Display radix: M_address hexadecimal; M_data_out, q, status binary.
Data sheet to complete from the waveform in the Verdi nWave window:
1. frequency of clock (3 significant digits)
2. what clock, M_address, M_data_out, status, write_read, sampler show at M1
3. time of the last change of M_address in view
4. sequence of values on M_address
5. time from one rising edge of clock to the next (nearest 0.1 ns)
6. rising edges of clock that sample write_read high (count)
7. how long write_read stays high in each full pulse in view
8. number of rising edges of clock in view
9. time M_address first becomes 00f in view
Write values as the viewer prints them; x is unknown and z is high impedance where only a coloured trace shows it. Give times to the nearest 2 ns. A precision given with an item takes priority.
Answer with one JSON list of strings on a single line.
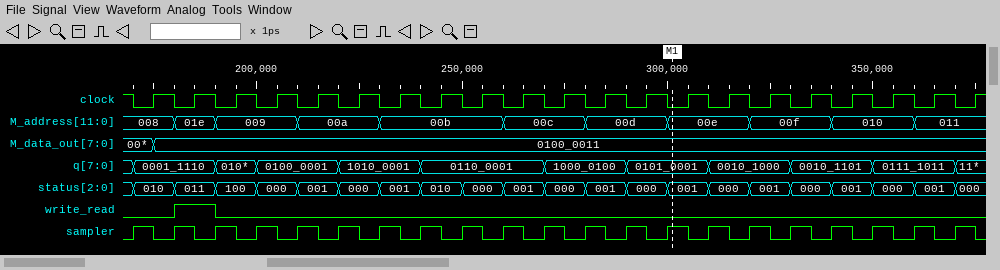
["100 MHz", "clock=0, M_address=00e, M_data_out=0100_0011, status=001, write_read=0, sampler=1", "360 ns", "008, 01e, 009, 00a, 00b, 00c, 00d, 00e, 00f, 010, 011", "10 ns", "1", "10 ns", "21", "320 ns"]
